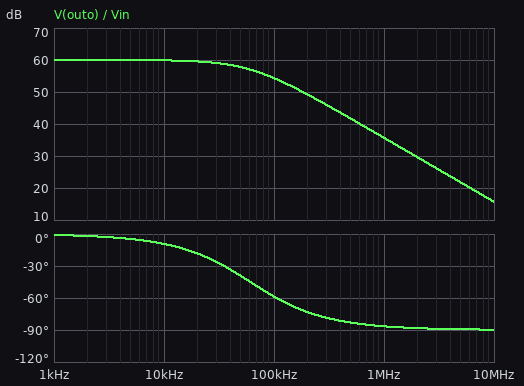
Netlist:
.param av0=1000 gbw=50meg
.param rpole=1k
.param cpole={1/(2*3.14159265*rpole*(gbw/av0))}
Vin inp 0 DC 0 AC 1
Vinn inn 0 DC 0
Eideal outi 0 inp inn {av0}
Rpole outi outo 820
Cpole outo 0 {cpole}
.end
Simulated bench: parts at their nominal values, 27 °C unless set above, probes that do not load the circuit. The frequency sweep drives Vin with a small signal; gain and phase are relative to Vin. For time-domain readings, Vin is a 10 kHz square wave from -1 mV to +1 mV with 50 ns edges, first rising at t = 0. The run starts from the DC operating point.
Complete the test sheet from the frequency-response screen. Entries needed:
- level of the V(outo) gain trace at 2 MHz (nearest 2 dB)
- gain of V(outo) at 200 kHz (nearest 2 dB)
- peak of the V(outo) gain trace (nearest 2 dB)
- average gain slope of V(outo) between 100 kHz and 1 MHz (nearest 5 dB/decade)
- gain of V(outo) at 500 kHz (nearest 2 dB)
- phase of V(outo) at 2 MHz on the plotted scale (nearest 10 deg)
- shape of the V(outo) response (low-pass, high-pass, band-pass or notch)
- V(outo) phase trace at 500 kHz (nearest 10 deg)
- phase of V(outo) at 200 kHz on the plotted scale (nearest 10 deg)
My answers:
30 dB
50 dB
60 dB
-20 dB/decade
42 dB
-90 deg
low-pass
-80 deg
-70 deg
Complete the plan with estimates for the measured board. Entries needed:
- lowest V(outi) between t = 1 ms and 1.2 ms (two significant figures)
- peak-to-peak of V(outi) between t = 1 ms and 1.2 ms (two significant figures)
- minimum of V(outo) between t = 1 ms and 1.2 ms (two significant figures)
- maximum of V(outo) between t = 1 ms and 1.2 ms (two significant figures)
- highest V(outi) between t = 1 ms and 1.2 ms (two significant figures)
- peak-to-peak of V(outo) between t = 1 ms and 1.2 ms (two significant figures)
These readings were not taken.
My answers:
-1.0 V
2.0 V
-1.0 V
1.0 V
1.0 V
2.0 V
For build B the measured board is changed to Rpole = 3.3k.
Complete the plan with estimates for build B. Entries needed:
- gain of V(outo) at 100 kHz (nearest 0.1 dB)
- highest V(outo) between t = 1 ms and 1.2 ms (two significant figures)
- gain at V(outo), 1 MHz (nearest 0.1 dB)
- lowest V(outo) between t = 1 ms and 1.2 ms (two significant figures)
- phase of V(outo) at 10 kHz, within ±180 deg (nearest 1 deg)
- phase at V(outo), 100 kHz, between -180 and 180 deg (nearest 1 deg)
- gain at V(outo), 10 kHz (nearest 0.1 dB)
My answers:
43.5 dB
980 mV
23.6 dB
-980 mV
-33 deg
-81 deg
58.4 dB
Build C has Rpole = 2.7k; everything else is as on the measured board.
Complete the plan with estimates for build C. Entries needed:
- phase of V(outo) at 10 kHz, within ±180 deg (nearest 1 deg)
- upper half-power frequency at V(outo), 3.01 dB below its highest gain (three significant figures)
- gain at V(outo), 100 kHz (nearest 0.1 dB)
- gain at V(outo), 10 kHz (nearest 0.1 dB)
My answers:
-28 deg
18.5 kHz
45.2 dB
58.9 dB
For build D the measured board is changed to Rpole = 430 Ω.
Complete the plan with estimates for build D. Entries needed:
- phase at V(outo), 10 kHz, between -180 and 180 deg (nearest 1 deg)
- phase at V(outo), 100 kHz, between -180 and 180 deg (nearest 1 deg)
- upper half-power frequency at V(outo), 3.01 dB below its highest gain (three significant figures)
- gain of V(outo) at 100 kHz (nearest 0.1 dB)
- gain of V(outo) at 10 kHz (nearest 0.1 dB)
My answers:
-5 deg
-41 deg
116 kHz
57.6 dB
60.0 dB
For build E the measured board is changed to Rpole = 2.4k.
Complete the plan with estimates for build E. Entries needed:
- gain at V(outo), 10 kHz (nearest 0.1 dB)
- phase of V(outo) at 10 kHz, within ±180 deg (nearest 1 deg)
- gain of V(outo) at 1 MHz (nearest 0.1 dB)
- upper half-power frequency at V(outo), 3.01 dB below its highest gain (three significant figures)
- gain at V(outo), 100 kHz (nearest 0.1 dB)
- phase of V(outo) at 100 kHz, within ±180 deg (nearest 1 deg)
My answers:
59.1 dB
-26 deg
26.4 dB
20.8 kHz
46.2 dB
-78 deg
